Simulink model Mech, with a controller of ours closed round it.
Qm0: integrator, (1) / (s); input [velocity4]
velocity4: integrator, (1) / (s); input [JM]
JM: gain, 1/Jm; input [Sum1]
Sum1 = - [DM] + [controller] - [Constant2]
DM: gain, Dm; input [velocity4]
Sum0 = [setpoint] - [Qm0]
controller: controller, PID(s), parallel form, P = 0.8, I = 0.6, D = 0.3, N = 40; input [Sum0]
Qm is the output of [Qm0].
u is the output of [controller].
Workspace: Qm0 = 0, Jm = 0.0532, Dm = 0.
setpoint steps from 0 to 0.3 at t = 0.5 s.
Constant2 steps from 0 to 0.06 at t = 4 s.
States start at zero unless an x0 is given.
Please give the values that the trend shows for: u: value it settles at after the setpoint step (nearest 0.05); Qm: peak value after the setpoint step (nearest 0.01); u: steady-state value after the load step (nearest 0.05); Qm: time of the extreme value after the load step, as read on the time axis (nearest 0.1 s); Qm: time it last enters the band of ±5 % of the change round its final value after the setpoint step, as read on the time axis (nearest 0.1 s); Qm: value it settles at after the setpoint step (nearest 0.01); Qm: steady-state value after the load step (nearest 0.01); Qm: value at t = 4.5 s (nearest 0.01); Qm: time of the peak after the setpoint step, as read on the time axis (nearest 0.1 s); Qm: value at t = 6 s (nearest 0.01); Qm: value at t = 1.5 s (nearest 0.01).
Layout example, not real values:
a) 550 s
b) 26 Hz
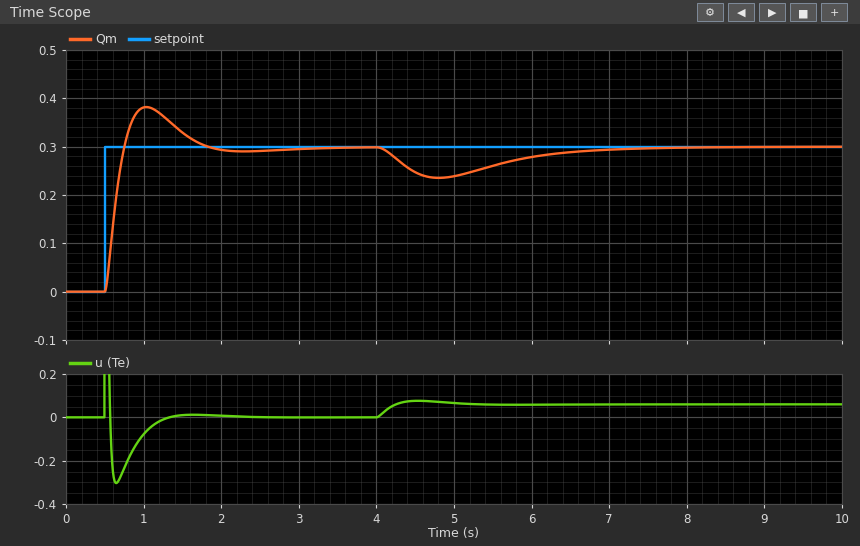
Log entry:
a) 0.00
b) 0.38
c) 0.05
d) 4.8 s
e) 1.6 s
f) 0.30
g) 0.30
h) 0.25
i) 1.0 s
j) 0.28
k) 0.33
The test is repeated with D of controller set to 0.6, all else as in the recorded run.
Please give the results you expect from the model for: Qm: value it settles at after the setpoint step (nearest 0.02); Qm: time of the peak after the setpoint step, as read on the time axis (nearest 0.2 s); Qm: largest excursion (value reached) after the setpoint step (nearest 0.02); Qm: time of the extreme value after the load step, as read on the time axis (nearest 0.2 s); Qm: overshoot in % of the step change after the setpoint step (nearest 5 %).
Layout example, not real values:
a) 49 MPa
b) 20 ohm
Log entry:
a) 0.30
b) 0.8 s
c) 0.34
d) 5.2 s
e) 10 %
